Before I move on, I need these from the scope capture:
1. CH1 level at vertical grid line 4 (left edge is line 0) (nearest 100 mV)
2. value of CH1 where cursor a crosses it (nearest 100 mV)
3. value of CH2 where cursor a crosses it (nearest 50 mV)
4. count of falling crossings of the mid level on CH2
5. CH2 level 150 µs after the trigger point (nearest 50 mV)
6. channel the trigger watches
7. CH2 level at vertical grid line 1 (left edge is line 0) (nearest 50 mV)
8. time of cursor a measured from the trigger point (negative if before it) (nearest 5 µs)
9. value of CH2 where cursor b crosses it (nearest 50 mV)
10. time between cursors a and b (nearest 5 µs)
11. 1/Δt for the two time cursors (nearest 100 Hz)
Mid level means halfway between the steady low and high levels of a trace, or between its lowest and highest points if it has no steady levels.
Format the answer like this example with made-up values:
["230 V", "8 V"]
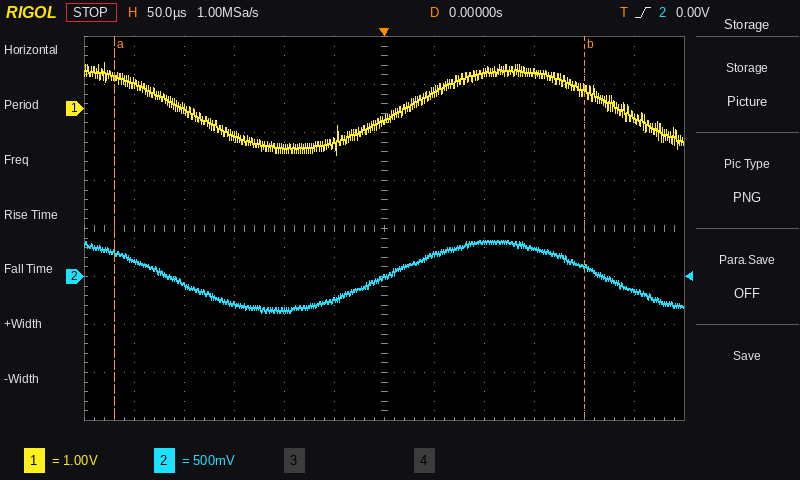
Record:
["-800 mV", "700 mV", "250 mV", "2", "300 mV", "CH2", "150 mV", "-270 µs", "100 mV", "470 µs", "2.1 kHz"]
